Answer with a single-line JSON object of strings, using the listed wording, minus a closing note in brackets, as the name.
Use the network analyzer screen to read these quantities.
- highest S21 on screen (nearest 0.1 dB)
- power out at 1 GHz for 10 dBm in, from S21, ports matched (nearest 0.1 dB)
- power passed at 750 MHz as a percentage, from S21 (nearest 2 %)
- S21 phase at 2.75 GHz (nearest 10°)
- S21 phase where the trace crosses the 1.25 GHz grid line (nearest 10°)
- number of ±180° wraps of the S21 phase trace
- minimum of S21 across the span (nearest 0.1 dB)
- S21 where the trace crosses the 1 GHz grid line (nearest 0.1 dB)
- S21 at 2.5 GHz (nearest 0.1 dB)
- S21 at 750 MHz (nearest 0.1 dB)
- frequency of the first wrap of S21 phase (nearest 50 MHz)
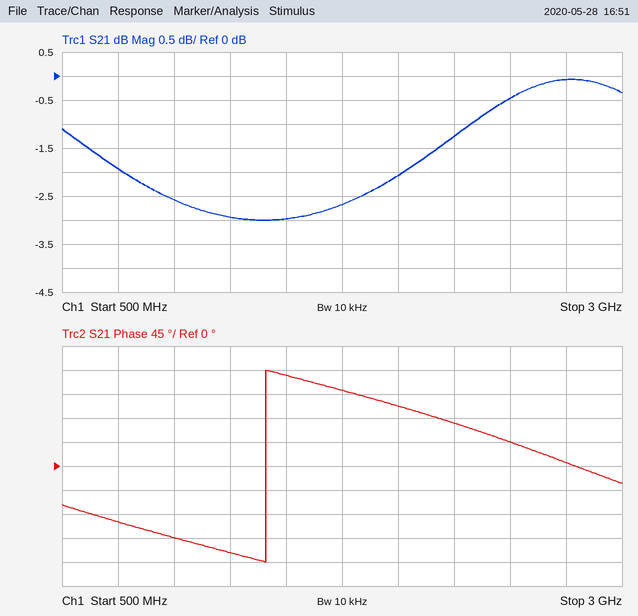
{"highest S21 on screen": "-0.1 dB", "power out at 1 GHz for 10 dBm in, from S21, ports matched": "7.4 dBm", "power passed at 750 MHz as a percentage, from S21": "64 %", "S21 phase at 2.75 GHz": "10°", "S21 phase where the trace crosses the 1.25 GHz grid line": "-160°", "number of ±180° wraps of the S21 phase trace": "1", "minimum of S21 across the span": "-3.0 dB", "S21 where the trace crosses the 1 GHz grid line": "-2.6 dB", "S21 at 2.5 GHz": "-0.5 dB", "S21 at 750 MHz": "-1.9 dB", "frequency of the first wrap of S21 phase": "1.40 GHz"}
